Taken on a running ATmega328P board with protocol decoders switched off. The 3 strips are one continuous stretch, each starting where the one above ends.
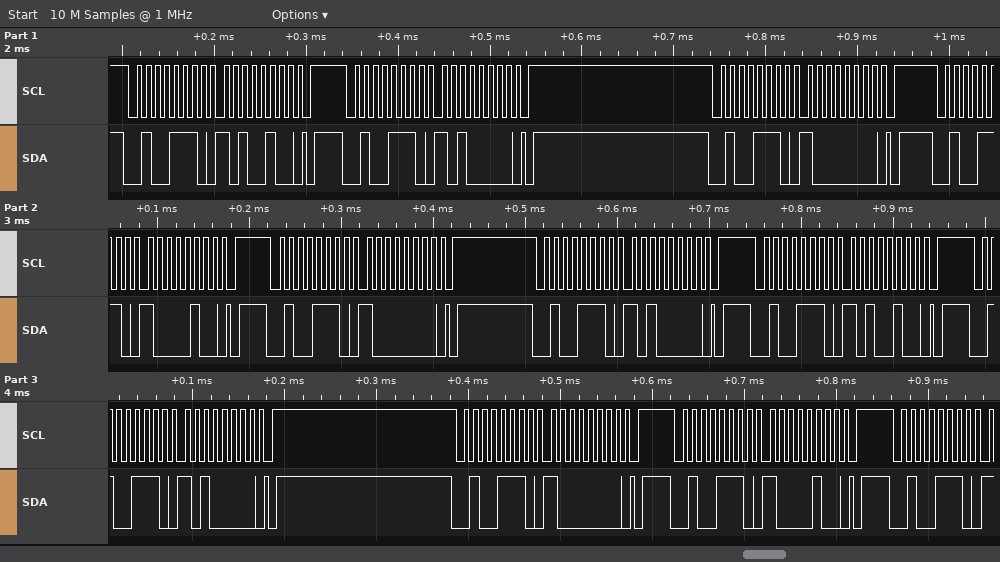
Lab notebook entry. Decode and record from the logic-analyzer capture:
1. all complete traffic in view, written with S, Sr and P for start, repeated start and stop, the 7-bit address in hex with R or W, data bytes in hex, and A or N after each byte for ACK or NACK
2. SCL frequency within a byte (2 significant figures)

S 27W A A4 A P S 27W A A0 A P S 27W A 80 A P S 27W A 84 A P S 27W A 80 A P S 27W A A0 A P S 27W A A4 A P S 27W A A0 A P S 27W A 80 A P S 27W A 84 A P S 27W A
100 kHz
